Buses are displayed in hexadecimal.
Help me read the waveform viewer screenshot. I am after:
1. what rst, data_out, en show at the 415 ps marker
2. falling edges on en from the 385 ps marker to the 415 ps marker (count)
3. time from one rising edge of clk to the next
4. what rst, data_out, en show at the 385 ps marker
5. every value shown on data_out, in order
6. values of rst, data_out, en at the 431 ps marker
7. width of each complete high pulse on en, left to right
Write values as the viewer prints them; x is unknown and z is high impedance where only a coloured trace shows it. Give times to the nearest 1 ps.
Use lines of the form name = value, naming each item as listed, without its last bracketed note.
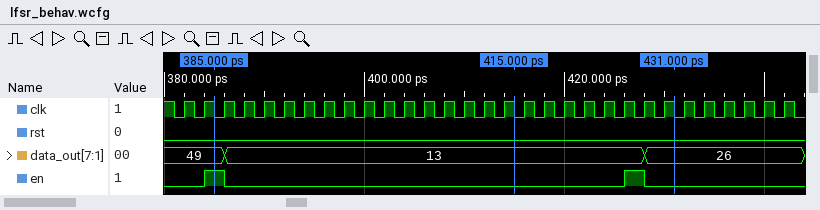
what rst, data_out, en show at the 415 ps marker = rst=0, data_out=13, en=0
falling edges on en from the 385 ps marker to the 415 ps marker = 1
time from one rising edge of clk to the next = 2 ps
what rst, data_out, en show at the 385 ps marker = rst=0, data_out=49, en=1
every value shown on data_out, in order = 49, 13, 26
values of rst, data_out, en at the 431 ps marker = rst=0, data_out=26, en=0
width of each complete high pulse on en, left to right = 2 ps, 2 ps
